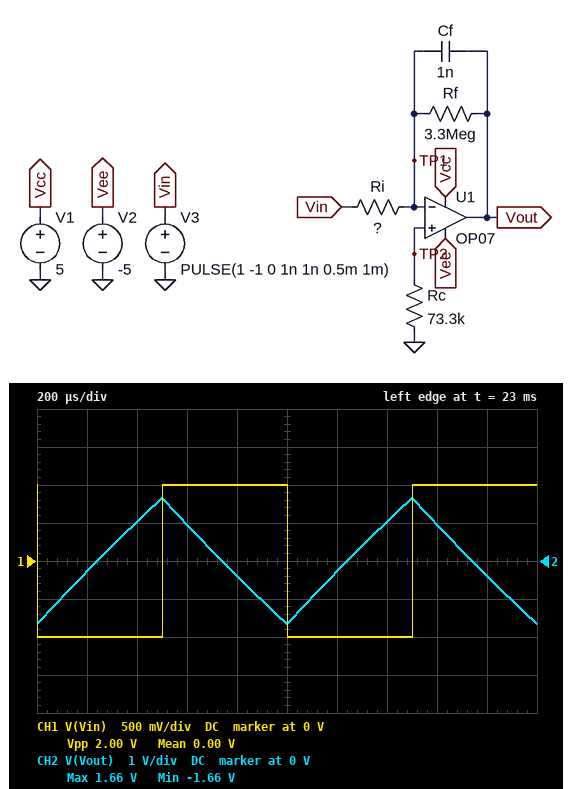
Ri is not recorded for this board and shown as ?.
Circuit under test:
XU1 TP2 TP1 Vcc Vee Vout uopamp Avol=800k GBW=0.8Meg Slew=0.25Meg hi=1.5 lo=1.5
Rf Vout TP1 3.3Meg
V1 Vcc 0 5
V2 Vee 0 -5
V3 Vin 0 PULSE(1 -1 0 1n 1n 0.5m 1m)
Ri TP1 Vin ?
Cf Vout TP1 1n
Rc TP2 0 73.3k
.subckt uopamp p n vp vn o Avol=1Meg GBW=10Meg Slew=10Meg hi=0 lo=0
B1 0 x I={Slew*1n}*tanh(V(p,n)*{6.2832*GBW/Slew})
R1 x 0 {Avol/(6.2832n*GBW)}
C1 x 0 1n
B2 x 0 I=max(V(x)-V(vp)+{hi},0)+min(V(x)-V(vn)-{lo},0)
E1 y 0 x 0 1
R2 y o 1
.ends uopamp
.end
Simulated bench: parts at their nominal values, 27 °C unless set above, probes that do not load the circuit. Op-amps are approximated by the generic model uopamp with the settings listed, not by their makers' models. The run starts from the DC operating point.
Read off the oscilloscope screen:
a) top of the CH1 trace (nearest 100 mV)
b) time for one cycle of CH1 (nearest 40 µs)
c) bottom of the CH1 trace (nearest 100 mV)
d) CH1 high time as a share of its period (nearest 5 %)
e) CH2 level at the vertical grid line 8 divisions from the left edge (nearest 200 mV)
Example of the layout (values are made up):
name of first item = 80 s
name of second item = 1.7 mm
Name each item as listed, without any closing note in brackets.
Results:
top of the CH1 trace = 1.0 V
time for one cycle of CH1 = 1.00 ms
bottom of the CH1 trace = -1.0 V
CH1 high time as a share of its period = 50 %
CH2 level at the vertical grid line 8 divisions from the left edge = 1.0 V
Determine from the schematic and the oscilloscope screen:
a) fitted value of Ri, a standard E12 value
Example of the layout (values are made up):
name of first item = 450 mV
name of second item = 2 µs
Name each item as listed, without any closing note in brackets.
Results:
fitted value of Ri, a standard E12 value = 150 kΩ
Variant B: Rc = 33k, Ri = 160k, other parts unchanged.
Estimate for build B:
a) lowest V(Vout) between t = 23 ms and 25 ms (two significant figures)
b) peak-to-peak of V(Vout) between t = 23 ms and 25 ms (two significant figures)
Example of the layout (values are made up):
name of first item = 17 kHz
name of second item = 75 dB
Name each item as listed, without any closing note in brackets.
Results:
lowest V(Vout) between t = 23 ms and 25 ms = -1.6 V
peak-to-peak of V(Vout) between t = 23 ms and 25 ms = 3.1 V
